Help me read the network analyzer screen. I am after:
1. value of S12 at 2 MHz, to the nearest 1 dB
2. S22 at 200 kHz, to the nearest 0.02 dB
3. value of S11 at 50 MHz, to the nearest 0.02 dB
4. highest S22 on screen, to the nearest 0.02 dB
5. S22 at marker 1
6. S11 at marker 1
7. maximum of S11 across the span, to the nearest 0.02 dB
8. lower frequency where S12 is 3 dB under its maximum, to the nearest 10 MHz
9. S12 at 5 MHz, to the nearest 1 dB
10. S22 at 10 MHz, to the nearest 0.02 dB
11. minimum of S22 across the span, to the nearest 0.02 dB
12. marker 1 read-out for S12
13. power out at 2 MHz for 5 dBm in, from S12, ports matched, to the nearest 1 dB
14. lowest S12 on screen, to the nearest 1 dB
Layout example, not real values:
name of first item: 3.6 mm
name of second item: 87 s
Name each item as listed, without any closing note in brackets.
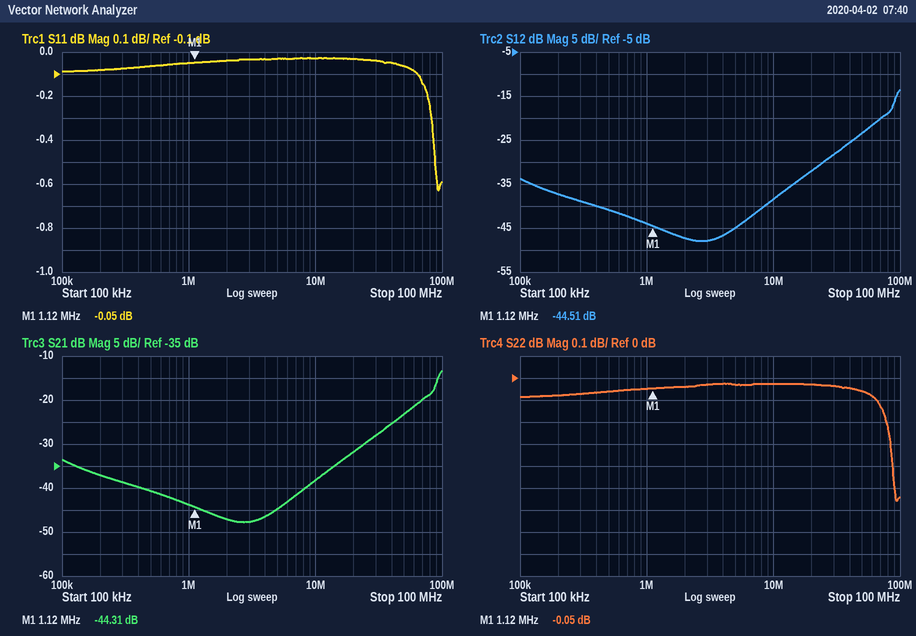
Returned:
value of S12 at 2 MHz, to the nearest 1 dB: -47 dB
S22 at 200 kHz, to the nearest 0.02 dB: -0.08 dB
value of S11 at 50 MHz, to the nearest 0.02 dB: -0.06 dB
highest S22 on screen, to the nearest 0.02 dB: -0.02 dB
S22 at marker 1: -0.05 dB
S11 at marker 1: -0.05 dB
maximum of S11 across the span, to the nearest 0.02 dB: -0.02 dB
lower frequency where S12 is 3 dB under its maximum, to the nearest 10 MHz: 90 MHz
S12 at 5 MHz, to the nearest 1 dB: -45 dB
S22 at 10 MHz, to the nearest 0.02 dB: -0.02 dB
minimum of S22 across the span, to the nearest 0.02 dB: -0.56 dB
marker 1 read-out for S12: -44.51 dB
power out at 2 MHz for 5 dBm in, from S12, ports matched, to the nearest 1 dB: -42 dBm
lowest S12 on screen, to the nearest 1 dB: -48 dB
